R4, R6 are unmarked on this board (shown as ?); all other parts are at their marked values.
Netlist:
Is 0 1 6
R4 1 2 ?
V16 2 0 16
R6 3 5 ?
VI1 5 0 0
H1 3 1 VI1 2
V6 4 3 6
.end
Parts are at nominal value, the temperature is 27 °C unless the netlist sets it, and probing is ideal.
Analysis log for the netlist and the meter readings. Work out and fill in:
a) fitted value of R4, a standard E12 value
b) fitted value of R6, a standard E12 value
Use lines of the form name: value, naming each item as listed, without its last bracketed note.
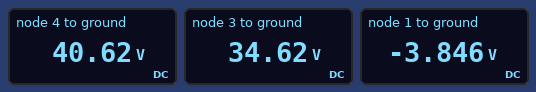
fitted value of R4, a standard E12 value: 1.5 Ω
fitted value of R6, a standard E12 value: 1.8 Ω
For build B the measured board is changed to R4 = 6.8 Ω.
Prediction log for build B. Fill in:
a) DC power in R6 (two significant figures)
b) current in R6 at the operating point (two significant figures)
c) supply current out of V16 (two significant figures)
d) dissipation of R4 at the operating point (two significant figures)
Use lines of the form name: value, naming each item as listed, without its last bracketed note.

DC power in R6: 130 W
current in R6 at the operating point: 8.6 A
supply current out of V16: 2.6 A
dissipation of R4 at the operating point: 46 W
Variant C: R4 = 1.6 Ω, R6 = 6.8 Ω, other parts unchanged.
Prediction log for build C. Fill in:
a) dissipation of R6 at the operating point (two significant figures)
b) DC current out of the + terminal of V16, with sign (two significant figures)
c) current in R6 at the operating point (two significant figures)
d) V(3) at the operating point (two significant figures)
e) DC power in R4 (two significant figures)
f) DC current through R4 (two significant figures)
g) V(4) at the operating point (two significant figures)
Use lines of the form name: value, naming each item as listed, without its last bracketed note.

dissipation of R6 at the operating point: 110 W
DC current out of the + terminal of V16, with sign: -2.0 A
current in R6 at the operating point: 4.0 A
V(3) at the operating point: 27 V
DC power in R4: 6.4 W
DC current through R4: 2.0 A
V(4) at the operating point: 33 V
